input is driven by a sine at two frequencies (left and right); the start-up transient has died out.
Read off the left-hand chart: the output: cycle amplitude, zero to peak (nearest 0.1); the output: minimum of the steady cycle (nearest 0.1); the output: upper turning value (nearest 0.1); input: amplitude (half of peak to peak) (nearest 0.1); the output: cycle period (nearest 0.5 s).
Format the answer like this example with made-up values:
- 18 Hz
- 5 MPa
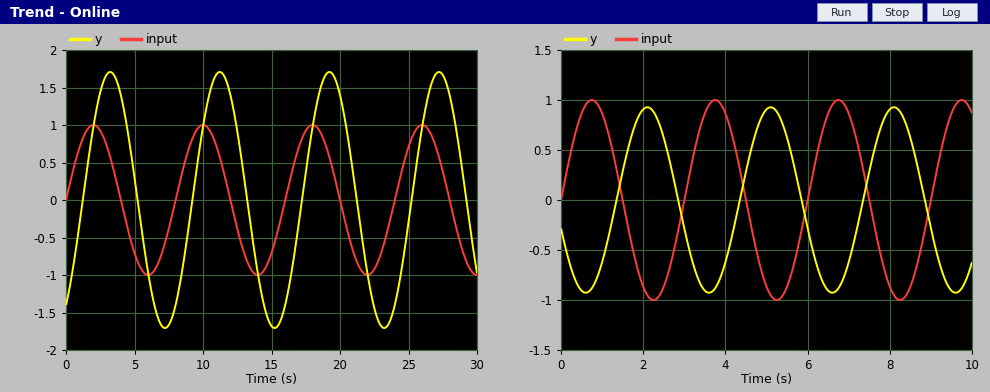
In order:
- 1.7
- -1.7
- 1.7
- 1.0
- 8.0 s
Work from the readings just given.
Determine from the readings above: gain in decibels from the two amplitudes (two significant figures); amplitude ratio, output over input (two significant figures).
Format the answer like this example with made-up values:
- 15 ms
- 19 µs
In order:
- 4.6 dB
- 1.7
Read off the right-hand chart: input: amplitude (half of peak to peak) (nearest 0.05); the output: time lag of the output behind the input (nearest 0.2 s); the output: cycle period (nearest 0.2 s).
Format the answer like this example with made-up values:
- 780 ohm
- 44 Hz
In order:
- 1.00
- 1.4 s
- 3.0 s
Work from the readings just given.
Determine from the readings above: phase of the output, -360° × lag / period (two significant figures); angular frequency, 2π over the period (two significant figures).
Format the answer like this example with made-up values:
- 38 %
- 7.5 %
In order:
- -170°
- 2.1 rad/s
